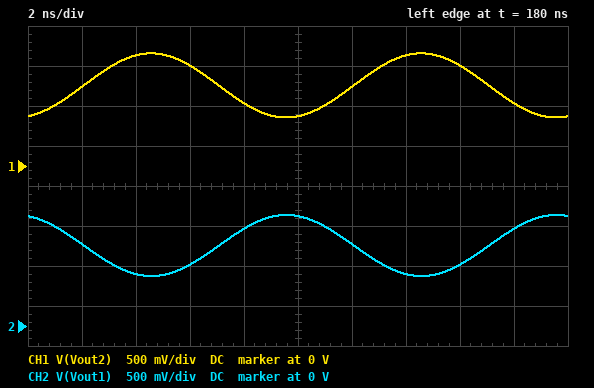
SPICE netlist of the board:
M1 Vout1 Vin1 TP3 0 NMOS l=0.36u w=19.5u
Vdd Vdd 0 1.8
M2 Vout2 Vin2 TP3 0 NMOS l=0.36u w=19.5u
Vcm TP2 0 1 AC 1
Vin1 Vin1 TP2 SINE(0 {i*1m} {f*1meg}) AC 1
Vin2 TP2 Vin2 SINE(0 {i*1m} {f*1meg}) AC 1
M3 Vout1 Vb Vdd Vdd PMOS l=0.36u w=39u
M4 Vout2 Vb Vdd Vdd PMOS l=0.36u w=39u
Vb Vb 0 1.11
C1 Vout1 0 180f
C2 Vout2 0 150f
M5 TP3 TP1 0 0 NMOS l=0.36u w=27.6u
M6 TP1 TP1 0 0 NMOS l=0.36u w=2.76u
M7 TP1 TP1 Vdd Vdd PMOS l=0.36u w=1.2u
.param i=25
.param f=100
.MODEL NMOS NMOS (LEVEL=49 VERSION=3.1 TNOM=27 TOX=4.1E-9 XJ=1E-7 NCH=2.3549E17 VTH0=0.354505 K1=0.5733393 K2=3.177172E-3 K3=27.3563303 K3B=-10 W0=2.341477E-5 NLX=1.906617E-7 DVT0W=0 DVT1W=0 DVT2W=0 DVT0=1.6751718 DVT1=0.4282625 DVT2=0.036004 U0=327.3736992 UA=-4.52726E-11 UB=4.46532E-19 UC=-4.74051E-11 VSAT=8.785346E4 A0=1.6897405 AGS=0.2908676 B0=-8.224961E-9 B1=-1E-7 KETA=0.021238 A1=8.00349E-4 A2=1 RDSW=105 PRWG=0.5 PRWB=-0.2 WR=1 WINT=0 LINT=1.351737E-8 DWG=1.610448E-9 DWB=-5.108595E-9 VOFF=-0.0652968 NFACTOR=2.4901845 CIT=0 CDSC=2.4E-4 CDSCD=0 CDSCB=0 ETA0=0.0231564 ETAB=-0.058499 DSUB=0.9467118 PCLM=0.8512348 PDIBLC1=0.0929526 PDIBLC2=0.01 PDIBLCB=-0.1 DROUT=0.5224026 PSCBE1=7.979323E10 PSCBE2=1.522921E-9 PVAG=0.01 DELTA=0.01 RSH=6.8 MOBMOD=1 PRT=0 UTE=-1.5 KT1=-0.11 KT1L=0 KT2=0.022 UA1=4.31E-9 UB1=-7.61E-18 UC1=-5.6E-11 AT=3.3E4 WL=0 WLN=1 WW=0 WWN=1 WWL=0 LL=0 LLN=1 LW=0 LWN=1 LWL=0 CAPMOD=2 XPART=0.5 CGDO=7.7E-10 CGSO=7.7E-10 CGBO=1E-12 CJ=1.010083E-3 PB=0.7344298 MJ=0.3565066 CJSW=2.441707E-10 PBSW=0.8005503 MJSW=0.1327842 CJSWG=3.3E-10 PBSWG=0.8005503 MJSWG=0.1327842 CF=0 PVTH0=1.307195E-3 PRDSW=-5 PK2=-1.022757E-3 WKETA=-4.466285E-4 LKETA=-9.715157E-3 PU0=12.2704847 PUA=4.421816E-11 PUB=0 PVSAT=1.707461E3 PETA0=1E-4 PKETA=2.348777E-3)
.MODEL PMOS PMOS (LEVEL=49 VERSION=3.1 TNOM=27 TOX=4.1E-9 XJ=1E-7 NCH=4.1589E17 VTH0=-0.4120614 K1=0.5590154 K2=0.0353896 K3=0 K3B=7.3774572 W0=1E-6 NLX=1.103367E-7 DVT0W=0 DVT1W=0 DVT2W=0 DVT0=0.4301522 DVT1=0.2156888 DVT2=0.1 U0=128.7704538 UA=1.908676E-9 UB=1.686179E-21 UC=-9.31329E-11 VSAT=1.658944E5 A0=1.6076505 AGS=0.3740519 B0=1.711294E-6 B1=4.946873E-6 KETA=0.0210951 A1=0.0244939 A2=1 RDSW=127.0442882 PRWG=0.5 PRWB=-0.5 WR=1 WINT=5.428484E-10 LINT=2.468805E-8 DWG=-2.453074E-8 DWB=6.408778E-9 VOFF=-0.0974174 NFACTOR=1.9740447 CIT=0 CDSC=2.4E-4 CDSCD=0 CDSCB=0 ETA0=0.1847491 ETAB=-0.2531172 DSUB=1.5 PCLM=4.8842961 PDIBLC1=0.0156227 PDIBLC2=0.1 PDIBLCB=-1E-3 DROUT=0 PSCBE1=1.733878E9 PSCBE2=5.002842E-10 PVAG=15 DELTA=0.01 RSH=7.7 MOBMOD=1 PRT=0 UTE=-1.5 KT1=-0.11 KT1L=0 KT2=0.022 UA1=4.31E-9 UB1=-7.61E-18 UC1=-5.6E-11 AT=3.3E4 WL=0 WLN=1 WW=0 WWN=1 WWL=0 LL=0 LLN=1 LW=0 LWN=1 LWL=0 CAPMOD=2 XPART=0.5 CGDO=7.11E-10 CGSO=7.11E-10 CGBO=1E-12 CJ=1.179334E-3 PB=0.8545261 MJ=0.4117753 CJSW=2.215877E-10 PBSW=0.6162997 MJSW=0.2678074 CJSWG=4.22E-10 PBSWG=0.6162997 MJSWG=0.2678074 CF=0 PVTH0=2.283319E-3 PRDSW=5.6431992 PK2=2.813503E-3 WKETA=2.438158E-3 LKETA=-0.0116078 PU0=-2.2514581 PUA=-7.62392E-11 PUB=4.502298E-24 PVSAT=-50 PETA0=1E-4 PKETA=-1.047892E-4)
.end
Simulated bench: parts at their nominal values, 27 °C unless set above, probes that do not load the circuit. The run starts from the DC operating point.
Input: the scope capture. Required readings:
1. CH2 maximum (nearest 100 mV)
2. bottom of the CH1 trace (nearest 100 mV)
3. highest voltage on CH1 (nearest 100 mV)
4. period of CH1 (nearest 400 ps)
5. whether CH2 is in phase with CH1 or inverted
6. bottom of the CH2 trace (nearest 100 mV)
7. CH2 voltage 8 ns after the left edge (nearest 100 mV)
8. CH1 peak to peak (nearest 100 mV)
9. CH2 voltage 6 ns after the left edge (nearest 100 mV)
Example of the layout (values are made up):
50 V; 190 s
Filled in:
1.4 V; 600 mV; 1.4 V; 10.0 ns; inverted; 600 mV; 1.2 V; 800 mV; 800 mV
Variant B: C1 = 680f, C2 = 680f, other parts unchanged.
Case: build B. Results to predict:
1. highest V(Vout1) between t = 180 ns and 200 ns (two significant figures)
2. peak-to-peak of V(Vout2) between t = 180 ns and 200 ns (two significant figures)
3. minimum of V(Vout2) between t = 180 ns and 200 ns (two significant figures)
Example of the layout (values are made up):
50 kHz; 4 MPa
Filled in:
1.1 V; 240 mV; 890 mV
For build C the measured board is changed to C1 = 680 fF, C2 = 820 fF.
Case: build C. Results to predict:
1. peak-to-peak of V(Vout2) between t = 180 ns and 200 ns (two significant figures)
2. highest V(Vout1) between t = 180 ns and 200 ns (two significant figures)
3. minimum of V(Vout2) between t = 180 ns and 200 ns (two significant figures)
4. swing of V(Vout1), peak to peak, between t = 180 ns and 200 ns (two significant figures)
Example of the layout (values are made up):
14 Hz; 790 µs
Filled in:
200 mV; 1.1 V; 910 mV; 240 mV
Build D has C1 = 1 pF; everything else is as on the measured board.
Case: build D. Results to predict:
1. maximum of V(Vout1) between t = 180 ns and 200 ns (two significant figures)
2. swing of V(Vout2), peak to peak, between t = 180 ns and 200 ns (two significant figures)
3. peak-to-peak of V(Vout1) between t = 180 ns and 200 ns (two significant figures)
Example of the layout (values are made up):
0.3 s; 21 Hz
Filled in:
1.1 V; 810 mV; 170 mV
